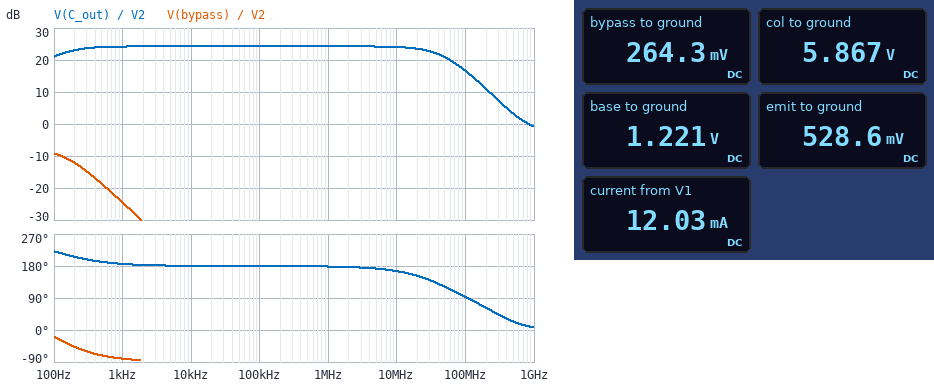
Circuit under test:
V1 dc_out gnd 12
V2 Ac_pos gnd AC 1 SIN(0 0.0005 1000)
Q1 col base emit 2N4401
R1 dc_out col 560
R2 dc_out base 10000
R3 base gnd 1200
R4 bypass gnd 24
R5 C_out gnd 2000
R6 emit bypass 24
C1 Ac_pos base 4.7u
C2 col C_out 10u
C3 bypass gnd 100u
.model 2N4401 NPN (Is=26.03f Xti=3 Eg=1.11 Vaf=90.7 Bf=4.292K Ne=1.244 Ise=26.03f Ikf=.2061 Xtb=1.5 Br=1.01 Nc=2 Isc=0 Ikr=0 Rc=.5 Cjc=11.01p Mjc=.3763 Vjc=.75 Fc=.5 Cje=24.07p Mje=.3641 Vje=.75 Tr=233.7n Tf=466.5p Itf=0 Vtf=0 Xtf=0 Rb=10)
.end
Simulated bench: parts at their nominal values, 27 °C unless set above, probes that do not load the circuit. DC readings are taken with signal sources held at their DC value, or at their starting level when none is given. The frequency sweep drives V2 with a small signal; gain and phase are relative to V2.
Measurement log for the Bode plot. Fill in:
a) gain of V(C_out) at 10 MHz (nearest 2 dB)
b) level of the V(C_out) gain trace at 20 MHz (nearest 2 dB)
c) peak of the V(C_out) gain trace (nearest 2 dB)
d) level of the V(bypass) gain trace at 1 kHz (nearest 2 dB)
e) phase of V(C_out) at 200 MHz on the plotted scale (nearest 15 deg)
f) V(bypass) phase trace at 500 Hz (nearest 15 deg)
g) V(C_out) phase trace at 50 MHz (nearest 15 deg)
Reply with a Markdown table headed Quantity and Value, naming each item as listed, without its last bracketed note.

| Quantity | Value |
|---|---|
| gain of V(C_out) at 10 MHz | 24 dB |
| level of the V(C_out) gain trace at 20 MHz | 24 dB |
| peak of the V(C_out) gain trace | 24 dB |
| level of the V(bypass) gain trace at 1 kHz | -24 dB |
| phase of V(C_out) at 200 MHz on the plotted scale | 60 deg |
| V(bypass) phase trace at 500 Hz | -75 deg |
| V(C_out) phase trace at 50 MHz | 120 deg |
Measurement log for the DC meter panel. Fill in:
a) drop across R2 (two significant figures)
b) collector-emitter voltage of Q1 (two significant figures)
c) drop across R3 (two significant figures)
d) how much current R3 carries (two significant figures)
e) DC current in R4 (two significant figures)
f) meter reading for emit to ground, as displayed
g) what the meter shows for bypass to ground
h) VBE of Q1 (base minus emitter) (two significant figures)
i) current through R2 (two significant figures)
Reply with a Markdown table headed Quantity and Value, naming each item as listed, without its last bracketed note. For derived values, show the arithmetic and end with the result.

| Quantity | Value |
|---|---|
| drop across R2 | 12 V - 1.221 V = 11 V |
| collector-emitter voltage of Q1 | 5.867 V - 528.6 mV = 5.3 V |
| drop across R3 | 1.221 V = 1.2 V |
| how much current R3 carries | (1.221 V) / 1.2 kΩ = 1.0 mA |
| DC current in R4 | (264.3 mV) / 24 Ω = 11 mA |
| meter reading for emit to ground, as displayed | 528.6 mV |
| what the meter shows for bypass to ground | 264.3 mV |
| VBE of Q1 (base minus emitter) | 1.221 V - 528.6 mV = 690 mV |
| current through R2 | (12 V - 1.221 V) / 10 kΩ = 1.1 mA |
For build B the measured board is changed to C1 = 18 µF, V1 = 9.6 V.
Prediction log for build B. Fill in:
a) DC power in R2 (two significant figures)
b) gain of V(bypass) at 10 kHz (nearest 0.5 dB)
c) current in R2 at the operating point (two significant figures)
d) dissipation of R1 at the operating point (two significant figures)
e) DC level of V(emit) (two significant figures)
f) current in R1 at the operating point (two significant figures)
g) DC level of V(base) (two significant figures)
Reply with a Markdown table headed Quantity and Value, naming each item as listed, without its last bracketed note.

| Quantity | Value |
|---|---|
| DC power in R2 | 7.4 mW |
| gain of V(bypass) at 10 kHz | -45.0 dB |
| current in R2 at the operating point | 860 µA |
| dissipation of R1 at the operating point | 23 mW |
| DC level of V(emit) | 310 mV |
| current in R1 at the operating point | 6.4 mA |
| DC level of V(base) | 990 mV |
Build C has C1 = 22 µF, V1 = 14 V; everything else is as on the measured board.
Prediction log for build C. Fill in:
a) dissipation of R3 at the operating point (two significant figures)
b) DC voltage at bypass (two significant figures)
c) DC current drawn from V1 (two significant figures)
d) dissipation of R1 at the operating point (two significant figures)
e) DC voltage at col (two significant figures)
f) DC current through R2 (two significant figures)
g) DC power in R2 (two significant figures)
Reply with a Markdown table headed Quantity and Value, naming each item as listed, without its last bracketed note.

| Quantity | Value |
|---|---|
| dissipation of R3 at the operating point | 1.7 mW |
| DC voltage at bypass | 360 mV |
| DC current drawn from V1 | 16 mA |
| dissipation of R1 at the operating point | 120 mW |
| DC voltage at col | 5.7 V |
| DC current through R2 | 1.3 mA |
| DC power in R2 | 16 mW |
